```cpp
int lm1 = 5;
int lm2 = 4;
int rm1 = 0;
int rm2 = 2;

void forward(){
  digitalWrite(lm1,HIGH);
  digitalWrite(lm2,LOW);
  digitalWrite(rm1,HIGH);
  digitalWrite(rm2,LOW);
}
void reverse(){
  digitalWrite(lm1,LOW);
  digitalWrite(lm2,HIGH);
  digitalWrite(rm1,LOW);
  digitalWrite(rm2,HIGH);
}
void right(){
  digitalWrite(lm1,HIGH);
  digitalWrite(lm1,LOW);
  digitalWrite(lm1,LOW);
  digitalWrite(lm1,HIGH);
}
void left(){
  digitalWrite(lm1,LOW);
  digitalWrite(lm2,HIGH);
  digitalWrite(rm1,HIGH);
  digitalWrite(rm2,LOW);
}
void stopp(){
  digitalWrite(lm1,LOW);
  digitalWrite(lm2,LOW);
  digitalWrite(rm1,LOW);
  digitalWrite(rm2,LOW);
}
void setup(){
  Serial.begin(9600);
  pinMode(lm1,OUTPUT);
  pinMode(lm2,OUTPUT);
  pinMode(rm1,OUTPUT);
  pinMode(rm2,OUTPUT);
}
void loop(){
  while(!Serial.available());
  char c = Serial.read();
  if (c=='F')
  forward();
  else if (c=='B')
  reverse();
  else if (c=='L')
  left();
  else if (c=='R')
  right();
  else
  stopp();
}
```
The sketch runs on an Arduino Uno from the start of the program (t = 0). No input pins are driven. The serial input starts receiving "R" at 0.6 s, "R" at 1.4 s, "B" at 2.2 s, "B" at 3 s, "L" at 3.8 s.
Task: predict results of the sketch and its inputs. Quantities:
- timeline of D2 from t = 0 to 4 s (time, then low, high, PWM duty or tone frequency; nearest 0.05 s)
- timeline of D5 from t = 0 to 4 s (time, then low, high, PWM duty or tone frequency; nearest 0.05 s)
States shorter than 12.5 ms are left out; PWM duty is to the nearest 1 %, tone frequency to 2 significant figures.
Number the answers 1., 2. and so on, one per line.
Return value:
1. 0 s low; 2.2 s high; 3.8 s low
2. 0 s low; 0.6 s high; 2.2 s low
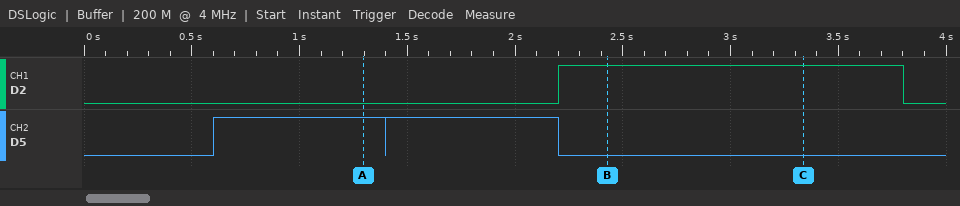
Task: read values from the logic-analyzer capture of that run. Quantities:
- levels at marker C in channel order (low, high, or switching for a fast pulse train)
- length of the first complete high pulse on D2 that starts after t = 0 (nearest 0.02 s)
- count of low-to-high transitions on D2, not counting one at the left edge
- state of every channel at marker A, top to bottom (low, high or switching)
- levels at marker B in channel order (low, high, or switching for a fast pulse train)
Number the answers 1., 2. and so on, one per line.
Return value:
1. D2 high, D5 low
2. 1.60 s
3. 1
4. D2 low, D5 high
5. D2 high, D5 low
